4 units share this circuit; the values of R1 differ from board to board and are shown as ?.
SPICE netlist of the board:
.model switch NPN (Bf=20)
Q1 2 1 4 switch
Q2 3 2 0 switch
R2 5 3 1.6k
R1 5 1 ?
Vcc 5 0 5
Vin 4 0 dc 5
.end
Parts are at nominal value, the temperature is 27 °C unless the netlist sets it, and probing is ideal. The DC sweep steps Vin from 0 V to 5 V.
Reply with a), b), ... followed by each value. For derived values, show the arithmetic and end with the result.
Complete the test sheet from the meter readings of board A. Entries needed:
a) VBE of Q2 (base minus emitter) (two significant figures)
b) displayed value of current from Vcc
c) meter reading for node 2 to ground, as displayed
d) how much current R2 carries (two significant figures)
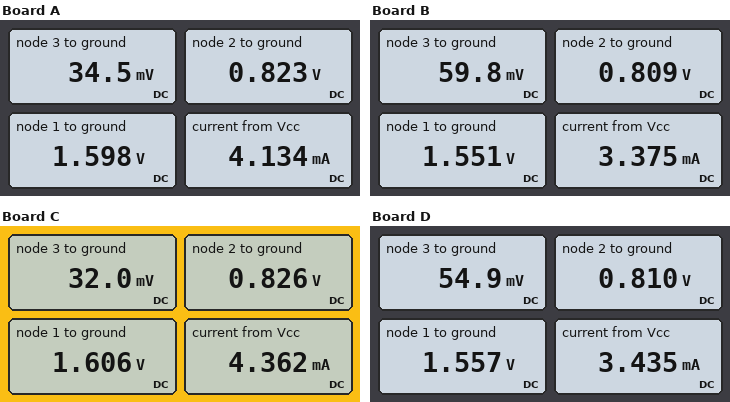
a) 823 mV = 820 mV
b) 4.134 mA
c) 0.823 V
d) (5 V - 34.5 mV) / 1.6 kΩ = 3.1 mA
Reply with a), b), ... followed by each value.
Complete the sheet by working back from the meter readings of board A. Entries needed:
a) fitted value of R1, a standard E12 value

a) 3.3 kΩ
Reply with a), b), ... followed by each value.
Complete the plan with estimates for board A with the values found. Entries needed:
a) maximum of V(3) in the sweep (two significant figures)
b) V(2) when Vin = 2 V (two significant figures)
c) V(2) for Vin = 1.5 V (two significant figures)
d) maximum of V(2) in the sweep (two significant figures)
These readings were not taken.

a) 5.0 V
b) 820 mV
c) 820 mV
d) 820 mV
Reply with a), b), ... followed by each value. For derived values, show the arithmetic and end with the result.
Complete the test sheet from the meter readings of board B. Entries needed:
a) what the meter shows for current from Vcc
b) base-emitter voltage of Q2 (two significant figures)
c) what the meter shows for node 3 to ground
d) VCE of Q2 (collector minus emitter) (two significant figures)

a) 3.375 mA
b) 809 mV = 810 mV
c) 59.8 mV
d) 59.8 mV = 60 mV
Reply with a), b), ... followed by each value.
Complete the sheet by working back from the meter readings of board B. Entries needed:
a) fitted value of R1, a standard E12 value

a) 12 kΩ
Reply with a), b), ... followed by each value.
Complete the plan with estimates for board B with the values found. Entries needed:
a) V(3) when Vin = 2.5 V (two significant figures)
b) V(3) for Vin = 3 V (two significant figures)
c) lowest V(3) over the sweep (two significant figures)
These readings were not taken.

a) 60 mV
b) 60 mV
c) 60 mV
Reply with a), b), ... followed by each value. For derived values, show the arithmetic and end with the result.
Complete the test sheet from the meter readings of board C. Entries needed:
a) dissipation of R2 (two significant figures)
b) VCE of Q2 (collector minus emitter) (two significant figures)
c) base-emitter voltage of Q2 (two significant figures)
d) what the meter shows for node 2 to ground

a) (5 V - 32 mV)^2 / 1.6 kΩ = 15 mW
b) 32 mV = 32 mV
c) 826 mV = 830 mV
d) 0.826 V
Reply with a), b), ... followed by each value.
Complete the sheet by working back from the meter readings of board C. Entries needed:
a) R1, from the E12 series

a) 2.7 kΩ
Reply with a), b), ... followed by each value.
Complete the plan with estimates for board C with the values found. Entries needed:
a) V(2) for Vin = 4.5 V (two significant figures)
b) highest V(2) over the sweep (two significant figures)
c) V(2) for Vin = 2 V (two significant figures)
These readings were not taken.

a) 830 mV
b) 830 mV
c) 830 mV
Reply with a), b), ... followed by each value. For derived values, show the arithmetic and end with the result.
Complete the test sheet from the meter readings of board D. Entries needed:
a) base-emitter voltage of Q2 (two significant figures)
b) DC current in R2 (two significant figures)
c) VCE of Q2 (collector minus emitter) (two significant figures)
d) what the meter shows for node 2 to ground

a) 810 mV = 810 mV
b) (5 V - 54.9 mV) / 1.6 kΩ = 3.1 mA
c) 54.9 mV = 55 mV
d) 0.810 V
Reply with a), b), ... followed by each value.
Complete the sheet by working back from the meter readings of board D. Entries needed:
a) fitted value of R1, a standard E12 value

a) 10 kΩ
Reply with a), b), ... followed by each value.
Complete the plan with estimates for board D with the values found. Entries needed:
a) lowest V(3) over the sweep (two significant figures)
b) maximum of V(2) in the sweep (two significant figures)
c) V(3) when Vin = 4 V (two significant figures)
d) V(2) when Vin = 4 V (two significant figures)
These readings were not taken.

a) 55 mV
b) 810 mV
c) 55 mV
d) 810 mV
